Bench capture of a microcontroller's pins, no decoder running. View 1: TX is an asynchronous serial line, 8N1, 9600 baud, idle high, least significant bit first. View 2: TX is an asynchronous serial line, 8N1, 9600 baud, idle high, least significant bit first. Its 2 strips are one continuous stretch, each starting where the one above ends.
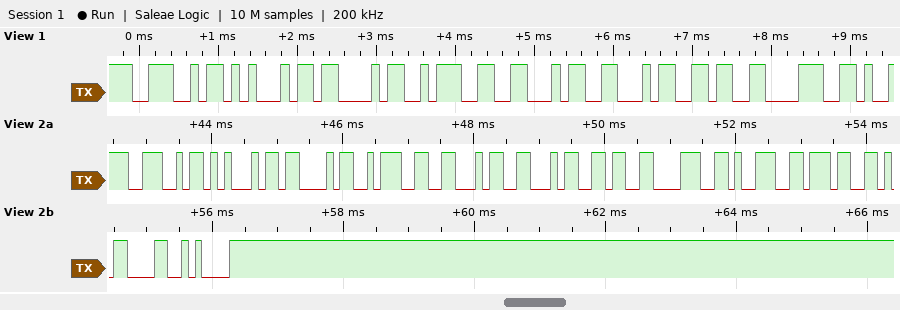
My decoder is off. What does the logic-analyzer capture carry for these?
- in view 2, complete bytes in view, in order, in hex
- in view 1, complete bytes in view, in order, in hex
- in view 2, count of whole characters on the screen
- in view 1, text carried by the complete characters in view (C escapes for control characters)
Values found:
0x4E 0x45 0x43 0x3A 0x46 0x46 0x36 0x38 0x39 0x37 0x0D 0x0A
4E 45 43 3A 46 46 36 38
12
"NEC:FF68"
